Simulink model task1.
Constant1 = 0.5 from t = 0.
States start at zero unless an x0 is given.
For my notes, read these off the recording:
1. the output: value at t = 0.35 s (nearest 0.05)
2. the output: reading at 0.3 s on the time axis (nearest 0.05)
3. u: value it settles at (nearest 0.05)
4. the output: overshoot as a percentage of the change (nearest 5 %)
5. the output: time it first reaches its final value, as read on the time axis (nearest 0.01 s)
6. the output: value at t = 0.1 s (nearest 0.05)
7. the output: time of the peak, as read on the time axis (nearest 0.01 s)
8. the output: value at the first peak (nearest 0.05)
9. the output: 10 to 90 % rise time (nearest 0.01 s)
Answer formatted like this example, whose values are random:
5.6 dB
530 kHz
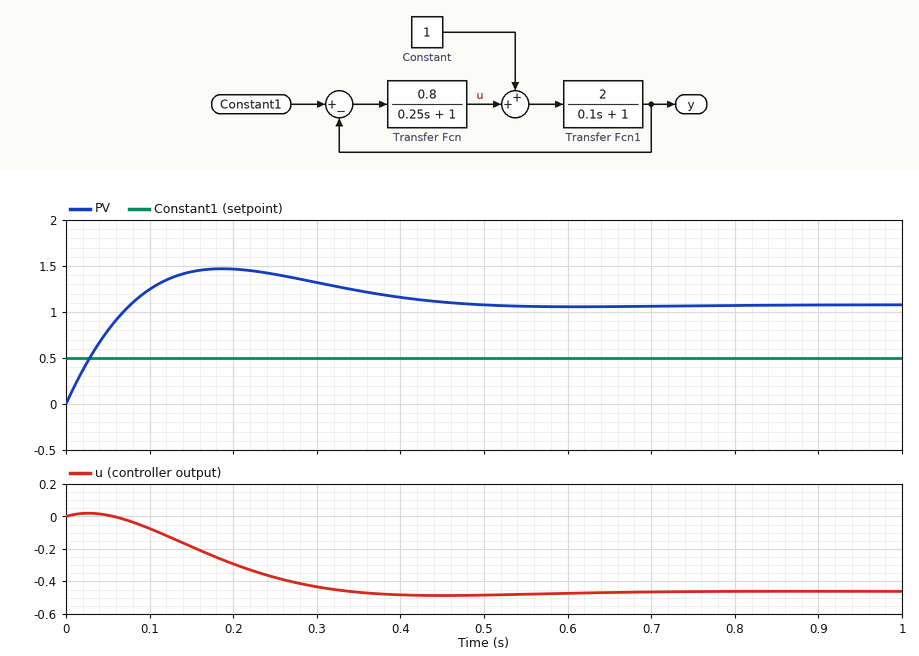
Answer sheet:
1.25
1.30
-0.45
35 %
0.08 s
1.25
0.19 s
1.45
0.06 s
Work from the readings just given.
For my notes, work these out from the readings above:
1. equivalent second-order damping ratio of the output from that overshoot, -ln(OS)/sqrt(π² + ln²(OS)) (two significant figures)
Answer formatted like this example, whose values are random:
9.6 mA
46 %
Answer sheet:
0.32
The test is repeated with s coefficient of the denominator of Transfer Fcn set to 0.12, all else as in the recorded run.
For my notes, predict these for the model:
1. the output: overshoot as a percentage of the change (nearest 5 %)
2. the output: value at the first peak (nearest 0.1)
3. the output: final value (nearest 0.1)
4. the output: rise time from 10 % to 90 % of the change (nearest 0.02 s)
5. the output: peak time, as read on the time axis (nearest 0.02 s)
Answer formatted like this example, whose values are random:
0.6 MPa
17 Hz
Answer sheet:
25 %
1.3
1.1
0.06 s
0.16 s
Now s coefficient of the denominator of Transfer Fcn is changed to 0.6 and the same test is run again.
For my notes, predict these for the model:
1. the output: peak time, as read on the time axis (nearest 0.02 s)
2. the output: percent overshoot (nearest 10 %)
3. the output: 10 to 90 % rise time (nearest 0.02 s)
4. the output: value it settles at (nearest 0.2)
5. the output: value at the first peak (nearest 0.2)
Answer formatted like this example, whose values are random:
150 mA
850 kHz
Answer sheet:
0.24 s
50 %
0.06 s
1.0
1.6
